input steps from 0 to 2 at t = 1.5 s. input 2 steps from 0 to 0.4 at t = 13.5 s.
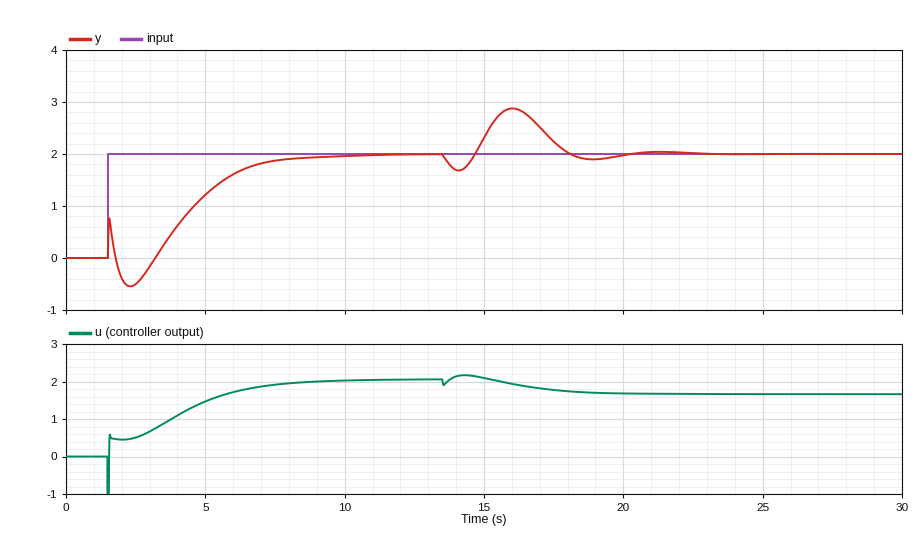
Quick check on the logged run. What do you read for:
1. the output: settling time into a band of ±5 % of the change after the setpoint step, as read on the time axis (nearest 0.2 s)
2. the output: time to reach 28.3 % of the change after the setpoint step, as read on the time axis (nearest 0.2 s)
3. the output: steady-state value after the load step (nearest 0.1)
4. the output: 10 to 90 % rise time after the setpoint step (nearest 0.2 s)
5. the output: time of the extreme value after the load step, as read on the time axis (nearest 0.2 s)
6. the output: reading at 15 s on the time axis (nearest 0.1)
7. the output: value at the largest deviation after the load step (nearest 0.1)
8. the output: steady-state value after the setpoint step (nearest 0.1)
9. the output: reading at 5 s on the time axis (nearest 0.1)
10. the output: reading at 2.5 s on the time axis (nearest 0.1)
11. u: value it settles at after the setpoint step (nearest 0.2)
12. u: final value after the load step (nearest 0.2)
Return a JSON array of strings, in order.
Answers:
["8.0 s", "1.6 s", "2.0", "5.4 s", "16.0 s", "2.3", "2.9", "2.0", "1.2", "-0.5", "2.0", "1.6"]
